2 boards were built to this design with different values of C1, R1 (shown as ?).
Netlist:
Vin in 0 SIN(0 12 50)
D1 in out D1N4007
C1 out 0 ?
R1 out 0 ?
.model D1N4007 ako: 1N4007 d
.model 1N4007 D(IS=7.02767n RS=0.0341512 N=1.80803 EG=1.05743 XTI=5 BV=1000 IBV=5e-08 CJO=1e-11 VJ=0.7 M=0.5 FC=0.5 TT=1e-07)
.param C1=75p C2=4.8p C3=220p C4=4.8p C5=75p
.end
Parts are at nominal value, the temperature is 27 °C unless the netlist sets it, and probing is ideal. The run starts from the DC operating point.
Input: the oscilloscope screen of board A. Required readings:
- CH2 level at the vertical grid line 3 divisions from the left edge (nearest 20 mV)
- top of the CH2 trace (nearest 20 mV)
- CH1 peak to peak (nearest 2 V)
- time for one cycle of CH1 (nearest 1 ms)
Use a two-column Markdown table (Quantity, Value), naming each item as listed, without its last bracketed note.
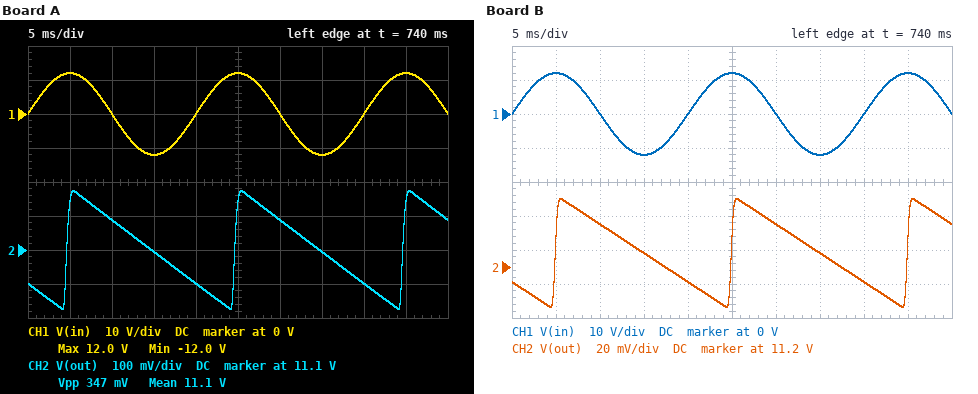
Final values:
| Quantity | Value |
|---|---|
| CH2 level at the vertical grid line 3 divisions from the left edge | 11.10 V |
| top of the CH2 trace | 11.28 V |
| CH1 peak to peak | 24 V |
| time for one cycle of CH1 | 20 ms |
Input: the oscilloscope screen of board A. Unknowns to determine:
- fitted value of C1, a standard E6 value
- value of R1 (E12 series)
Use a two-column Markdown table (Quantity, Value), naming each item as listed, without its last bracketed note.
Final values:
| Quantity | Value |
|---|---|
| fitted value of C1, a standard E6 value | 330 µF |
| value of R1 | 1.8 kΩ |
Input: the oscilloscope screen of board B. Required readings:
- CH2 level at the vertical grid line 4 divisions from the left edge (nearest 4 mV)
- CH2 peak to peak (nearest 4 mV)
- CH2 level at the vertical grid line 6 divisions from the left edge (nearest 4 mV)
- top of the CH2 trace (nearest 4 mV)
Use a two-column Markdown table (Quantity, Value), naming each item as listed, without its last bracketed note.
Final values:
| Quantity | Value |
|---|---|
| CH2 level at the vertical grid line 4 divisions from the left edge | 11.192 V |
| CH2 peak to peak | 64 mV |
| CH2 level at the vertical grid line 6 divisions from the left edge | 11.224 V |
| top of the CH2 trace | 11.240 V |
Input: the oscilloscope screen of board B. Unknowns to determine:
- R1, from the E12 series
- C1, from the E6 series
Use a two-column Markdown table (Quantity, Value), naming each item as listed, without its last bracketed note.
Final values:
| Quantity | Value |
|---|---|
| R1, from the E12 series | 3.3 kΩ |
| C1, from the E6 series | 1 mF |
